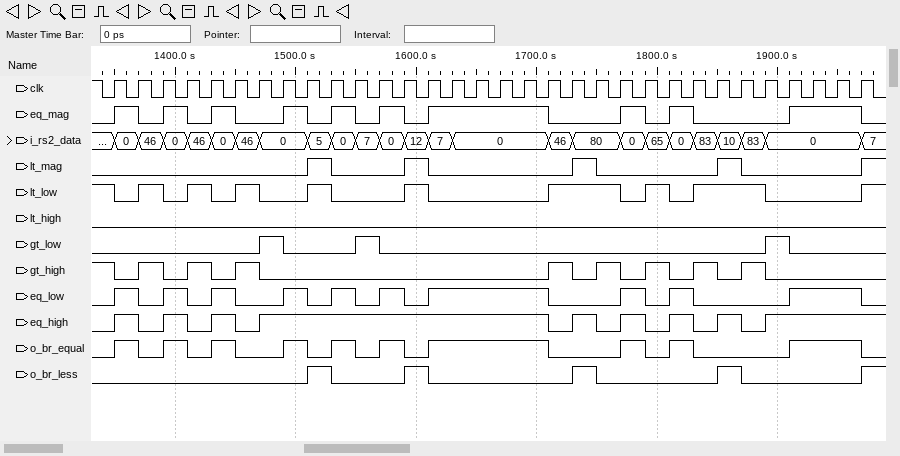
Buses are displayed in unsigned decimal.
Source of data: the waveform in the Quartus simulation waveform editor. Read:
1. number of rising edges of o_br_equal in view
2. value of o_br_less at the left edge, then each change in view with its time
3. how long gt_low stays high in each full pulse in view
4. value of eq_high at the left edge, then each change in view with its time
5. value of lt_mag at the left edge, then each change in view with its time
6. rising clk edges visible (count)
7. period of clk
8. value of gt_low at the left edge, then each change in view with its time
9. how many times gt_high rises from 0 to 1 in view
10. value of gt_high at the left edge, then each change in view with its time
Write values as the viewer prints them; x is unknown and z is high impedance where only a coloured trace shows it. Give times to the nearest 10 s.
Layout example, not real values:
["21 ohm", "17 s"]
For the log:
["10", "0, 1 at 1510 s, 0 at 1530 s, 1 at 1590 s, 0 at 1610 s, 1 at 1730 s, 0 at 1750 s, 1 at 1850 s, 0 at 1870 s, 1 at 1970 s", "20 s, 20 s, 20 s", "0, 1 at 1350 s, 0 at 1370 s, 1 at 1390 s, 0 at 1410 s, 1 at 1430 s, 0 at 1450 s, 1 at 1470 s, 0 at 1710 s, 1 at 1730 s, 0 at 1750 s, 1 at 1770 s, 0 at 1790 s, 1 at 1810 s, 0 at 1830 s, 1 at 1850 s, 0 at 1870 s, 1 at 1890 s", "0, 1 at 1510 s, 0 at 1530 s, 1 at 1590 s, 0 at 1610 s, 1 at 1730 s, 0 at 1750 s, 1 at 1850 s, 0 at 1870 s, 1 at 1970 s", "32", "20 s", "0, 1 at 1470 s, 0 at 1490 s, 1 at 1550 s, 0 at 1570 s, 1 at 1890 s, 0 at 1910 s", "8", "1, 0 at 1350 s, 1 at 1370 s, 0 at 1390 s, 1 at 1410 s, 0 at 1430 s, 1 at 1450 s, 0 at 1470 s, 1 at 1710 s, 0 at 1730 s, 1 at 1750 s, 0 at 1770 s, 1 at 1790 s, 0 at 1810 s, 1 at 1830 s, 0 at 1850 s, 1 at 1870 s, 0 at 1890 s"]
